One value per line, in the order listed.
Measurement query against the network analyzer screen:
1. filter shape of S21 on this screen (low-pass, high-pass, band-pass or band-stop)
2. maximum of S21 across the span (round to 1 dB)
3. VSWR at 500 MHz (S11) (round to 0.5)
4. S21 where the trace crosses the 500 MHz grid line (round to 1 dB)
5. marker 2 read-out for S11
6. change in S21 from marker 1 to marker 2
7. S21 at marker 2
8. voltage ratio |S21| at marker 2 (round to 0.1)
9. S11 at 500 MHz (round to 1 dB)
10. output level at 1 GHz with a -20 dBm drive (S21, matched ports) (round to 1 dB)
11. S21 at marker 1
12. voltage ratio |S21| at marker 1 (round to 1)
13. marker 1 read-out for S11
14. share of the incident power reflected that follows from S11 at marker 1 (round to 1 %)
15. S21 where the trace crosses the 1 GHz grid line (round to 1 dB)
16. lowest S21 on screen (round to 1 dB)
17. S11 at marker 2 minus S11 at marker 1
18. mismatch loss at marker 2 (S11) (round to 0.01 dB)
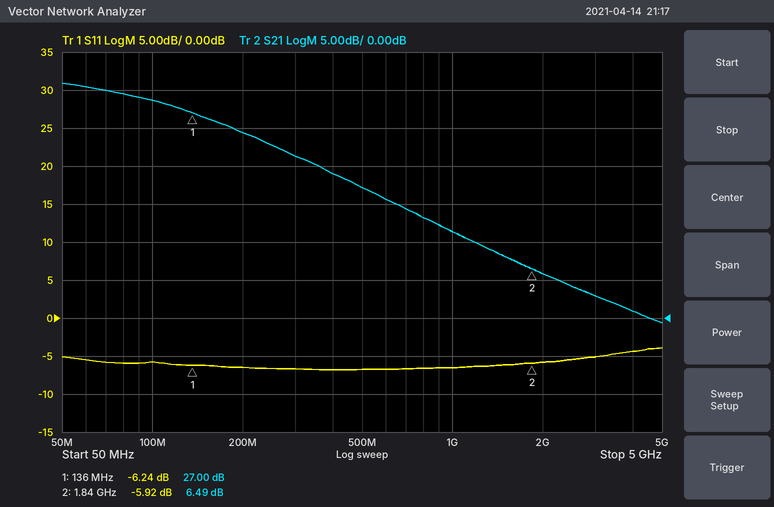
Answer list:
low-pass
31 dB
2.5
17 dB
-5.92 dB
-20.51 dB
6.49 dB
2.1
-7 dB
-9 dBm
27.00 dB
22
-6.24 dB
24 %
11 dB
-1 dB
0.32 dB
1.28 dB
